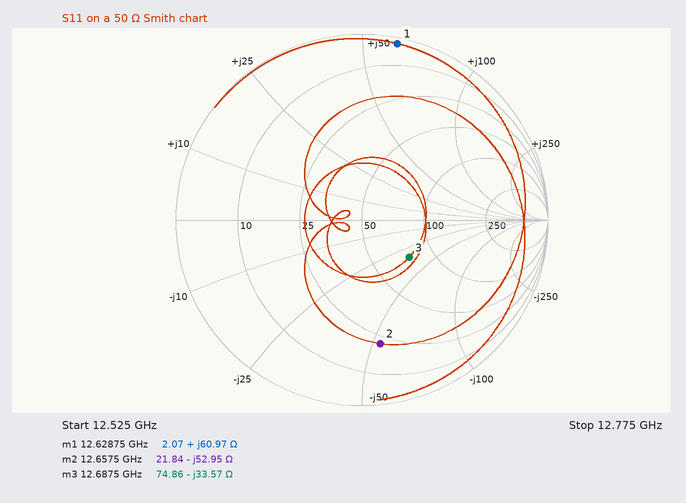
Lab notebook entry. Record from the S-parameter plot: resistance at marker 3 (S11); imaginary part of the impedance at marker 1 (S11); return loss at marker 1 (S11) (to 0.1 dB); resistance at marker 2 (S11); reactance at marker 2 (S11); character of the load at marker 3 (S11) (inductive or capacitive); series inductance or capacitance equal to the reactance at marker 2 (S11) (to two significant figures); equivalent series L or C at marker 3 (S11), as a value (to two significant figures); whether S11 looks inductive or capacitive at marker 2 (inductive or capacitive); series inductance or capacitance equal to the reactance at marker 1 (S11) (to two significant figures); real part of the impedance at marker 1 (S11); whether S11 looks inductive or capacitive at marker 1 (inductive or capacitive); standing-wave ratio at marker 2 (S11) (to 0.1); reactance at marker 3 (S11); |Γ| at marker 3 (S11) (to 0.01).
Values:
74.86 Ω
+60.97 Ω
0.3 dB
21.84 Ω
-52.95 Ω
capacitive
240 fF
370 fF
capacitive
770 pH
2.07 Ω
inductive
5.1
-33.57 Ω
0.32
